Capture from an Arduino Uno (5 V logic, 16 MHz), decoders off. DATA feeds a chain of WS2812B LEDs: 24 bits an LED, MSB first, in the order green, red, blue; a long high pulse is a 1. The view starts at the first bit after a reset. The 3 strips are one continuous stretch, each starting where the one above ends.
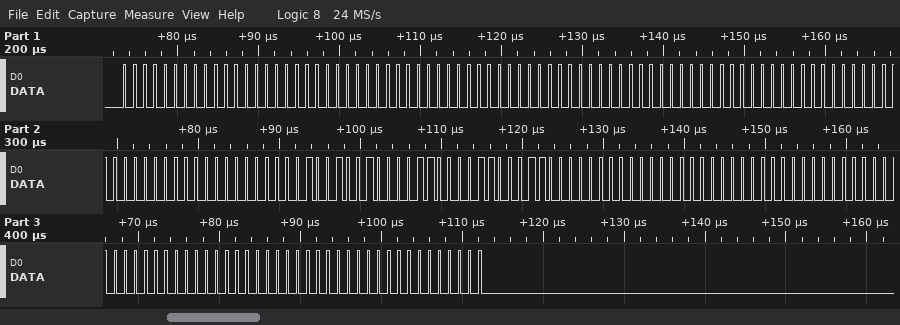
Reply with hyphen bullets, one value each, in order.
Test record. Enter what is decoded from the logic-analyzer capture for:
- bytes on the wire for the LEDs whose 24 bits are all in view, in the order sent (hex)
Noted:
- 00 00 00 00 00 00 00 00 00 00 00 00 92 18 63 00 00 00 00 00 00 00 00 00
